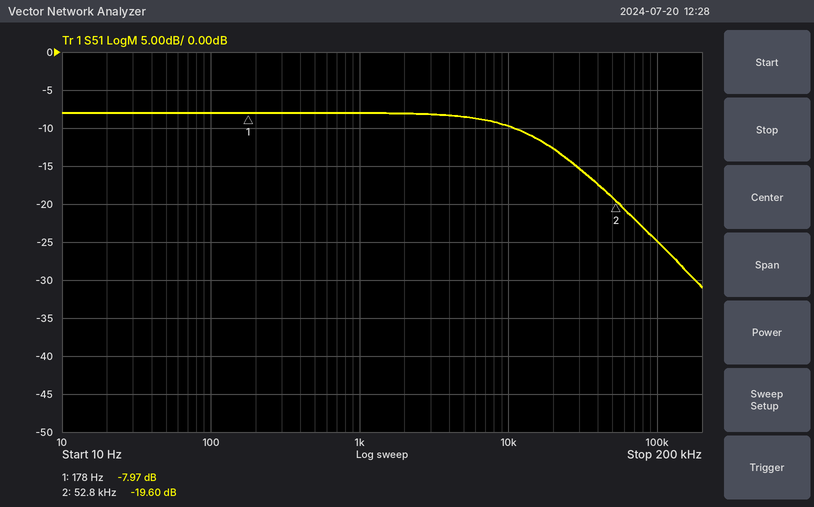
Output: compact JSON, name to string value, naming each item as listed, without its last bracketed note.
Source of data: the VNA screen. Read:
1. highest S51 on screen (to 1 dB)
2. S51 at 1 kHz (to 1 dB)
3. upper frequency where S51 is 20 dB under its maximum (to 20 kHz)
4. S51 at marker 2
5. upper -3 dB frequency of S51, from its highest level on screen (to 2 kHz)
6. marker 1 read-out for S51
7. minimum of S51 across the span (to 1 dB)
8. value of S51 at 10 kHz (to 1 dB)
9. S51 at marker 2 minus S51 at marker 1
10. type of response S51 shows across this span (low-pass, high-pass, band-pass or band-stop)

{"highest S51 on screen": "-8 dB", "S51 at 1 kHz": "-8 dB", "upper frequency where S51 is 20 dB under its maximum": "140 kHz", "S51 at marker 2": "-19.60 dB", "upper -3 dB frequency of S51, from its highest level on screen": "14 kHz", "marker 1 read-out for S51": "-7.97 dB", "minimum of S51 across the span": "-31 dB", "value of S51 at 10 kHz": "-10 dB", "S51 at marker 2 minus S51 at marker 1": "-11.63 dB", "type of response S51 shows across this span": "low-pass"}
